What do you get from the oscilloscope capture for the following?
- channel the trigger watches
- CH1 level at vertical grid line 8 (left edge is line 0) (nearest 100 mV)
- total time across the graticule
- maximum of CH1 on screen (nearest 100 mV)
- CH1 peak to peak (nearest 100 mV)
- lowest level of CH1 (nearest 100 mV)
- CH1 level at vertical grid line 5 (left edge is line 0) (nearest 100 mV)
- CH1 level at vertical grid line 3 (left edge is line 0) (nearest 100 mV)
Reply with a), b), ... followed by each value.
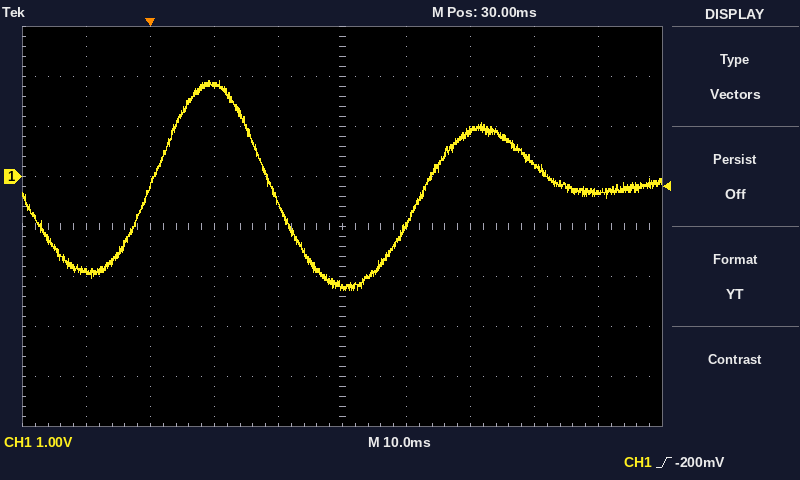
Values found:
a) CH1
b) 200 mV
c) 100 ms
d) 1.9 V
e) 4.2 V
f) -2.3 V
g) -2.2 V
h) 1.8 V
